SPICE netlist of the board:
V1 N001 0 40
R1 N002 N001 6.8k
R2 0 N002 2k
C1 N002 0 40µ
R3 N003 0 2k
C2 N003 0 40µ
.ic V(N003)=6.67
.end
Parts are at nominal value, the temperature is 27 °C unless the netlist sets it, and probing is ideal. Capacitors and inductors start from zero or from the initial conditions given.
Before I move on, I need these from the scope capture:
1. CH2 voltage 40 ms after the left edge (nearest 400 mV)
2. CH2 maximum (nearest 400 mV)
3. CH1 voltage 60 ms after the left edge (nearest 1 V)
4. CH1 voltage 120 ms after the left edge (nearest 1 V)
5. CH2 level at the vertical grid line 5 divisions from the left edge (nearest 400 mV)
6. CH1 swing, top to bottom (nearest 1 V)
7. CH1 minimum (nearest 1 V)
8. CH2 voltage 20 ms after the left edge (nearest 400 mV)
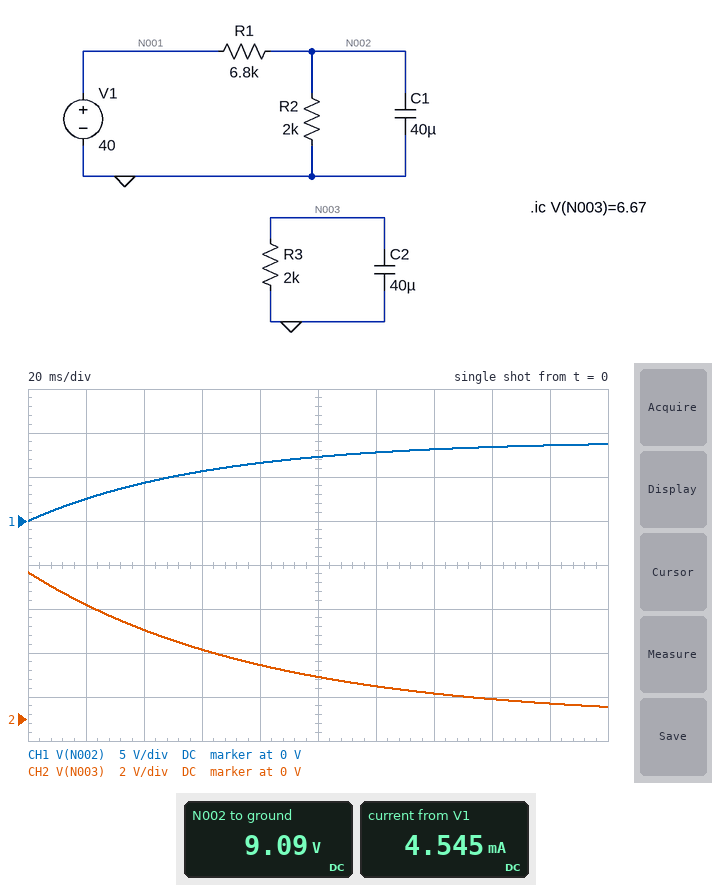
4.0 V
6.8 V
6 V
8 V
2.0 V
9 V
0 V
5.2 V
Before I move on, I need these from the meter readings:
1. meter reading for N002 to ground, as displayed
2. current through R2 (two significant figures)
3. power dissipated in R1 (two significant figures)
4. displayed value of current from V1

9.09 V
4.5 mA
140 mW
4.545 mA
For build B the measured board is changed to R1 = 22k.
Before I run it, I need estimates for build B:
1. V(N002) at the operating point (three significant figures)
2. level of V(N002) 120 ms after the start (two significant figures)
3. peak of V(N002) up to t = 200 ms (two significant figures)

3.33 V
2.7 V
3.1 V
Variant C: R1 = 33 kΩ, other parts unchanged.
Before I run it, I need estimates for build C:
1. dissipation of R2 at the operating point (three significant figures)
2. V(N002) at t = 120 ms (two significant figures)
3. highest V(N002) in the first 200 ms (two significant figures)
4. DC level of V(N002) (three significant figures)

2.61 mW
1.8 V
2.1 V
2.29 V
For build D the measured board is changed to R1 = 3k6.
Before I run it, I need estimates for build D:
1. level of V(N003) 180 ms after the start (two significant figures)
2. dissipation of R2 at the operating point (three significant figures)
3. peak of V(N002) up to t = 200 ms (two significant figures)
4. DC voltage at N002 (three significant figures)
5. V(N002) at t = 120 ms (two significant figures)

700 mV
102 mW
14 V
14.3 V
13 V
